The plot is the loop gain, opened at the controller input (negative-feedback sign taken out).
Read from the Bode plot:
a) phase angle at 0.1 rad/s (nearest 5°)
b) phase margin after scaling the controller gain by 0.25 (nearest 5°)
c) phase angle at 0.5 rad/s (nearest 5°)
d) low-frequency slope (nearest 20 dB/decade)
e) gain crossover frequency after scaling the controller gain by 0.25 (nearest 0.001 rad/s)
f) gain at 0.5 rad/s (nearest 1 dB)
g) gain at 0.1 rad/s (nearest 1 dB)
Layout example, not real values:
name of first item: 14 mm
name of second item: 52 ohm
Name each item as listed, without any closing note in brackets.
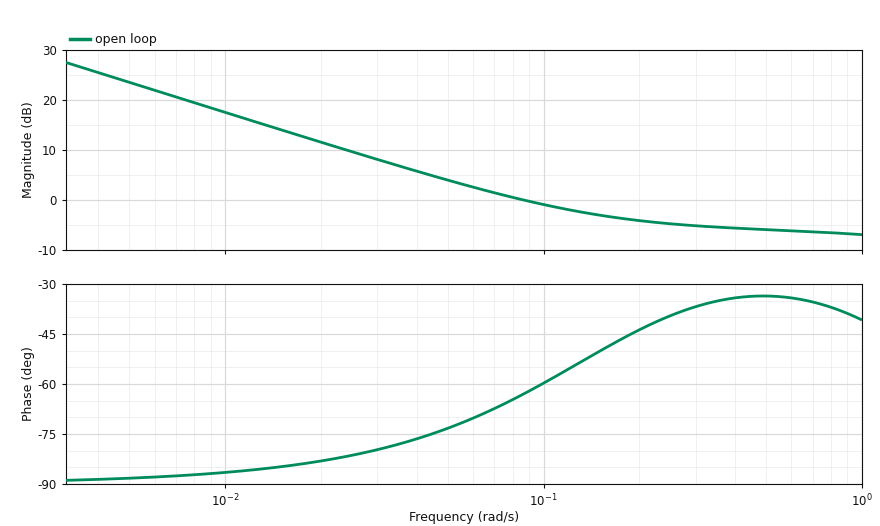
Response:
phase angle at 0.1 rad/s: -60°
phase margin after scaling the controller gain by 0.25: 95°
phase angle at 0.5 rad/s: -35°
low-frequency slope: -20 dB/decade
gain crossover frequency after scaling the controller gain by 0.25: 0.019 rad/s
gain at 0.5 rad/s: -6 dB
gain at 0.1 rad/s: -1 dB
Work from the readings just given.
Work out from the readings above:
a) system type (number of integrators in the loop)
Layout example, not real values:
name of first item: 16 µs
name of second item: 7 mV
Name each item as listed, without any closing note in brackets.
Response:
system type: 1
